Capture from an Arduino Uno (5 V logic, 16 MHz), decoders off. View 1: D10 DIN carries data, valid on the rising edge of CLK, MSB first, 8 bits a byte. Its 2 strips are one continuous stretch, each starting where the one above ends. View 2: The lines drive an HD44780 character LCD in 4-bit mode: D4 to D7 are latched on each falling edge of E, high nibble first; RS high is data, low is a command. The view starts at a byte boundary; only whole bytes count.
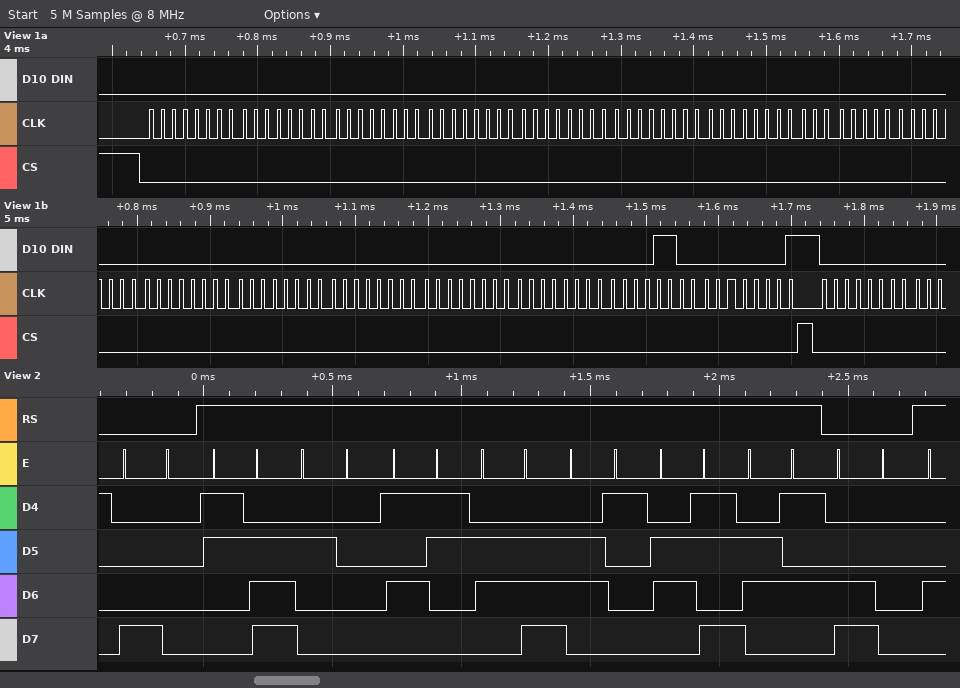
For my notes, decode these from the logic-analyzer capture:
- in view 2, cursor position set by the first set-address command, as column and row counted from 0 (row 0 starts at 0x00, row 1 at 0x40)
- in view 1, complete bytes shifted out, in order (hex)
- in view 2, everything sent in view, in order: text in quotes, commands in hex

column 0, row 0
00 00 00 00 00 00 00 00 00 00 00 00 00 00 0C 01 00
0x80 "> Snake" 0xC0
